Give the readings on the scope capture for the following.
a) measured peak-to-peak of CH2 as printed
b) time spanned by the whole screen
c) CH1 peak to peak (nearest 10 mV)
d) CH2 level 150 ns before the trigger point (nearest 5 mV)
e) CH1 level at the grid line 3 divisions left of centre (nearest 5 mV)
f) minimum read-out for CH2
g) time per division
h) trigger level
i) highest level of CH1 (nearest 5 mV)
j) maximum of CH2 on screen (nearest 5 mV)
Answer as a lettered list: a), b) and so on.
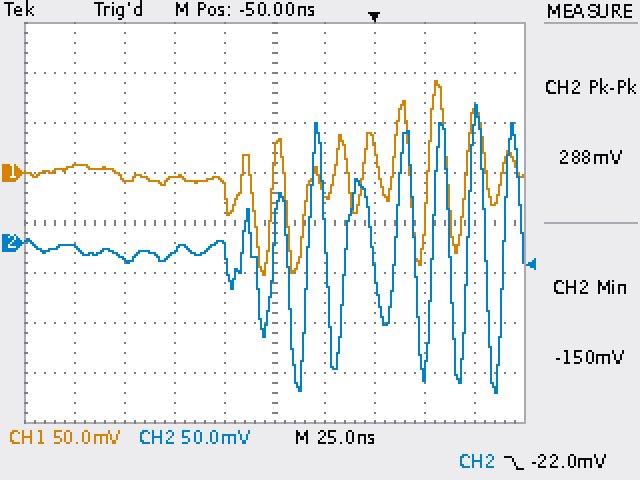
a) 288 mV
b) 250 ns
c) 190 mV
d) -5 mV
e) -5 mV
f) -150 mV
g) 25 ns
h) -22.0 mV
i) 90 mV
j) 140 mV
